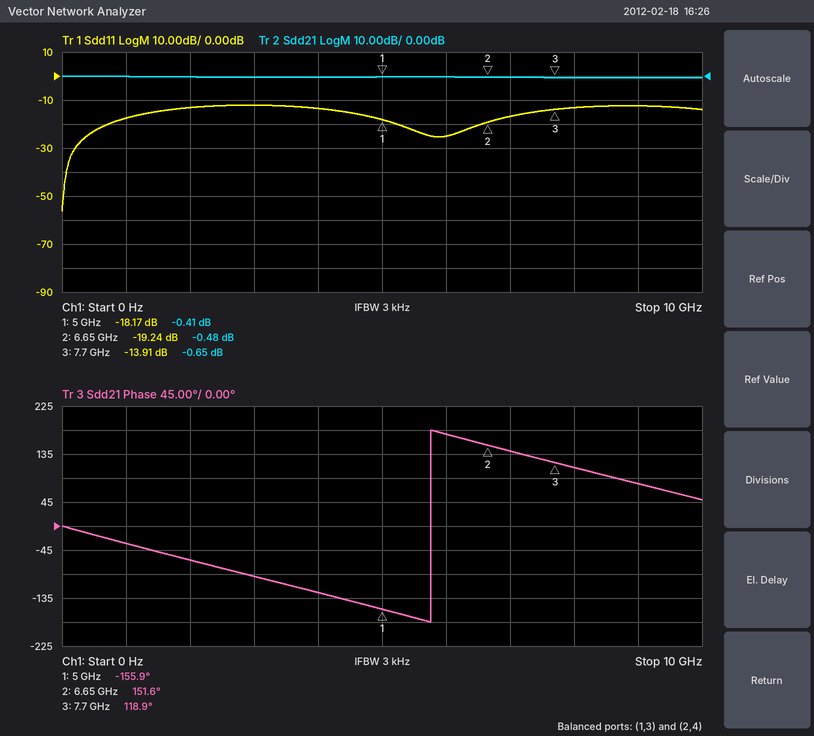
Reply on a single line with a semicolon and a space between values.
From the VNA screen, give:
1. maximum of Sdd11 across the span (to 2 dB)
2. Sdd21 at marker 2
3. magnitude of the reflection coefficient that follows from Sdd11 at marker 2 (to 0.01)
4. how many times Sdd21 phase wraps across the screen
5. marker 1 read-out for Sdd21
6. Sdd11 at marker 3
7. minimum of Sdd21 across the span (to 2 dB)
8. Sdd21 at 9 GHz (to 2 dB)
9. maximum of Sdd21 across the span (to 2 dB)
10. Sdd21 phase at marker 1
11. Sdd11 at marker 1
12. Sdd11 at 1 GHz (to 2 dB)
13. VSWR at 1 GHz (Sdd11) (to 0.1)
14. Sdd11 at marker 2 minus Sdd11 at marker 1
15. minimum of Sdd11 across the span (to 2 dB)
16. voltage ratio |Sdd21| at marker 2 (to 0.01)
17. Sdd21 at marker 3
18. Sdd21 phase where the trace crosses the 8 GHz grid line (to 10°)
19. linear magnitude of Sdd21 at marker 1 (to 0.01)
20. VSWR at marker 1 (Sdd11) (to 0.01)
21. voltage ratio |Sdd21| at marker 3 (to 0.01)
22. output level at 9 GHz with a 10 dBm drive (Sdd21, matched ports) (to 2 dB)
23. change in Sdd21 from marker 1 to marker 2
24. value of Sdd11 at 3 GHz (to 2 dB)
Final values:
-12 dB; -0.48 dB; 0.11; 1; -0.41 dB; -13.91 dB; 0 dB; 0 dB; 0 dB; -155.9°; -18.17 dB; -18 dB; 1.3; -1.07 dB; -56 dB; 0.95; -0.65 dB; 110°; 0.95; 1.28; 0.93; 10 dBm; -0.07 dB; -12 dB
